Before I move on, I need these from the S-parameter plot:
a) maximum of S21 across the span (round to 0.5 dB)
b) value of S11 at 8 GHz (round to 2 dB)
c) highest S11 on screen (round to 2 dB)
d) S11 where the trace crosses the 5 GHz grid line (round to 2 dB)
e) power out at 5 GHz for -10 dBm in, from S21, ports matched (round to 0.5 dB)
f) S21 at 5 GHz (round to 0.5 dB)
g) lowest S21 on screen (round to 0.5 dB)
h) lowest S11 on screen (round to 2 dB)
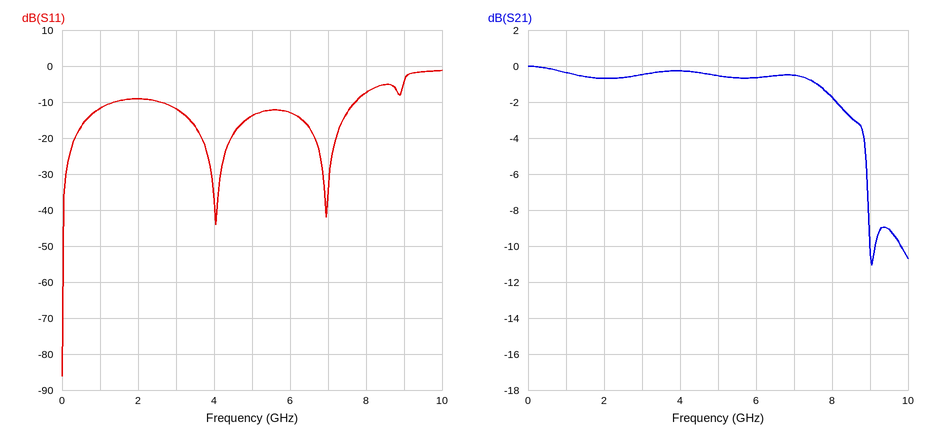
0.0 dB
-8 dB
-2 dB
-14 dB
-10.5 dBm
-0.5 dB
-11.0 dB
-86 dB
